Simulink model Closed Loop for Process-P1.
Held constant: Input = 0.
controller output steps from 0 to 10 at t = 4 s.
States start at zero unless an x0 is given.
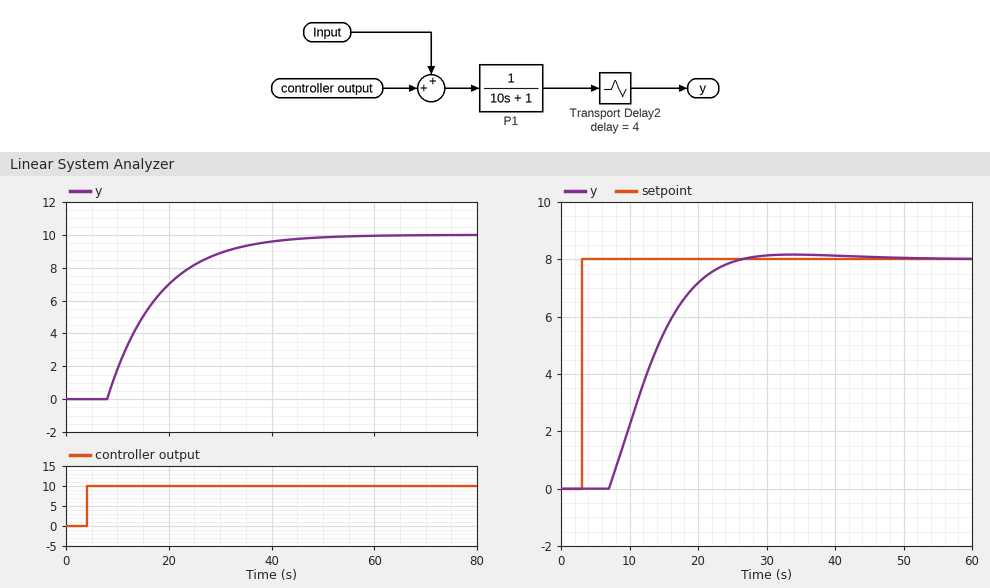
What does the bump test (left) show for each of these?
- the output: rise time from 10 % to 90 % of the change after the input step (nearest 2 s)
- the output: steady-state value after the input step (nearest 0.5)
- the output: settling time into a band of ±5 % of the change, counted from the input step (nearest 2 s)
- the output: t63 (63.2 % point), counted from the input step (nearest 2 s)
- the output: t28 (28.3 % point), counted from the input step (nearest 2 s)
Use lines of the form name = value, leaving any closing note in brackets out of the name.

the output: rise time from 10 % to 90 % of the change after the input step = 22 s
the output: steady-state value after the input step = 10.0
the output: settling time into a band of ±5 % of the change, counted from the input step = 34 s
the output: t63 (63.2 % point), counted from the input step = 14 s
the output: t28 (28.3 % point), counted from the input step = 8 s
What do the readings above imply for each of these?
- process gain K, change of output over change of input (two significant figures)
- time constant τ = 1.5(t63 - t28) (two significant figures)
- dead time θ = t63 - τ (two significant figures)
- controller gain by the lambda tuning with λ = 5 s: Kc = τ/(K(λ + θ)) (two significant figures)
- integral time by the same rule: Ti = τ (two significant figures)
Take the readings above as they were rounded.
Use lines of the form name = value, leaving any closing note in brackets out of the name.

process gain K, change of output over change of input = 1.0
time constant τ = 1.5(t63 - t28) = 9.0 s
dead time θ = t63 - τ = 5.0 s
controller gain by the lambda tuning with λ = 5 s: Kc = τ/(K(λ + θ)) = 0.90
integral time by the same rule: Ti = τ = 9.0 s
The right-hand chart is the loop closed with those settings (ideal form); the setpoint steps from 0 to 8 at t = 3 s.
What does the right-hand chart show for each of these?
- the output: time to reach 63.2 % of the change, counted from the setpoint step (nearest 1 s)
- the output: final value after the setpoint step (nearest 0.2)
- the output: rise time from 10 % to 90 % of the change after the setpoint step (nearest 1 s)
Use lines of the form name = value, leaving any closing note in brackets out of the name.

the output: time to reach 63.2 % of the change, counted from the setpoint step = 11 s
the output: final value after the setpoint step = 8.0
the output: rise time from 10 % to 90 % of the change after the setpoint step = 12 s
